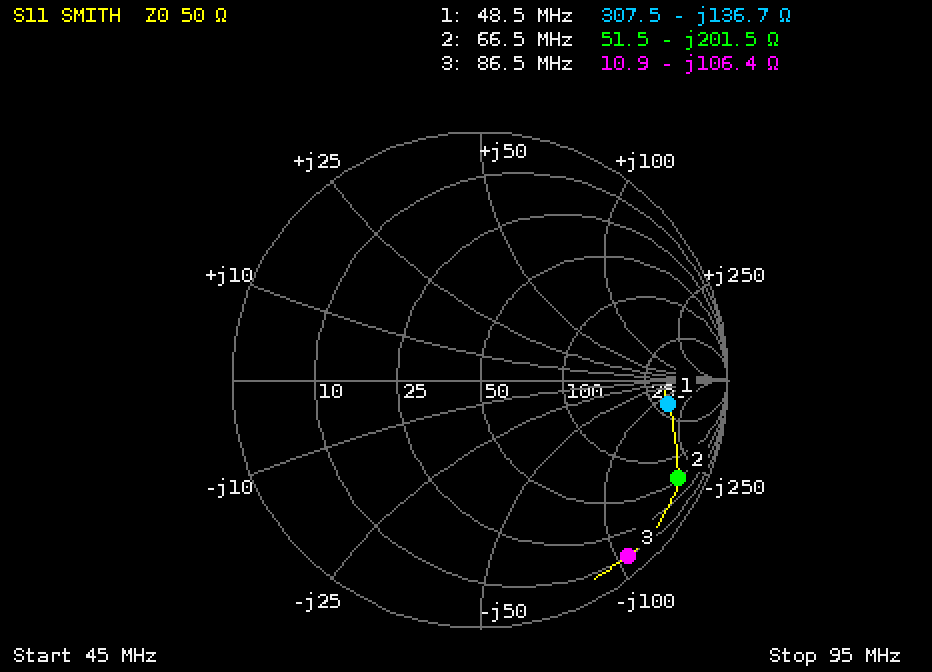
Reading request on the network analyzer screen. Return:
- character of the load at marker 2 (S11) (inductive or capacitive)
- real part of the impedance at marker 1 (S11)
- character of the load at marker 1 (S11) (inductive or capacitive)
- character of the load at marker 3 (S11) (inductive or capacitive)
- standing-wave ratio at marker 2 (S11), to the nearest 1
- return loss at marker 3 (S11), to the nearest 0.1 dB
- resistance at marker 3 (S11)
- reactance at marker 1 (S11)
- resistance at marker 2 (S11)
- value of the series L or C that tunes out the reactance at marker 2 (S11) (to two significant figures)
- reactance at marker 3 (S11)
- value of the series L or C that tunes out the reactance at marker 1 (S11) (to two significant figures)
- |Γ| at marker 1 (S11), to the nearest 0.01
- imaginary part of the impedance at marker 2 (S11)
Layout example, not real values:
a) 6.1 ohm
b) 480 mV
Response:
a) capacitive
b) 307.5 Ω
c) capacitive
d) capacitive
e) 18
f) 0.7 dB
g) 10.9 Ω
h) -136.7 Ω
i) 51.5 Ω
j) 480 nH
k) -106.4 Ω
l) 450 nH
m) 0.76
n) -201.5 Ω
